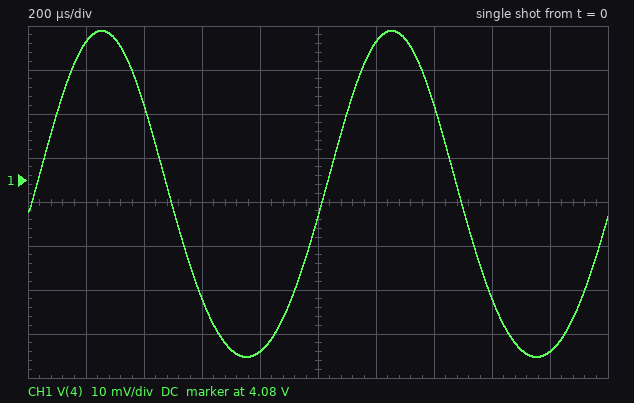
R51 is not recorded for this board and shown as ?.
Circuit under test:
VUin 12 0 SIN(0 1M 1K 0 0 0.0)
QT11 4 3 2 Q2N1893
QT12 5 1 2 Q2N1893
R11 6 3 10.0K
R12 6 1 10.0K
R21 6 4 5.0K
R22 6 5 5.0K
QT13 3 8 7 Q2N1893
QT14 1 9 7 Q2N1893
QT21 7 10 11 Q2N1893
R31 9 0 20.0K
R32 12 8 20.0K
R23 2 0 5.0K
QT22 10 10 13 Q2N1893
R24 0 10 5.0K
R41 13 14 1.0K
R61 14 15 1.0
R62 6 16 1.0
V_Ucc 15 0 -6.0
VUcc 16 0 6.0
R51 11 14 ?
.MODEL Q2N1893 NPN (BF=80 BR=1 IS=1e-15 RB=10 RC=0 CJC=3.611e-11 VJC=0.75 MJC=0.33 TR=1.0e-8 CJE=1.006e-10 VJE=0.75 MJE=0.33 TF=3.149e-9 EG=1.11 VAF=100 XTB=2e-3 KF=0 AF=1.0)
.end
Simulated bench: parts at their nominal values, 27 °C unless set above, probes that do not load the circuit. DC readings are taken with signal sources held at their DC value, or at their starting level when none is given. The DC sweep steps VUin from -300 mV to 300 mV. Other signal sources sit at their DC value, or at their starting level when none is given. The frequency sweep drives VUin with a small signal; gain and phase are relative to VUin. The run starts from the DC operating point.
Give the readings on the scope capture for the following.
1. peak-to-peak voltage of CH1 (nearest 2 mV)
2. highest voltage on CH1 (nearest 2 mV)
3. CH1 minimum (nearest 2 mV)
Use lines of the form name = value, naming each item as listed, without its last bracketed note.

peak-to-peak voltage of CH1 = 74 mV
highest voltage on CH1 = 4.114 V
CH1 minimum = 4.040 V
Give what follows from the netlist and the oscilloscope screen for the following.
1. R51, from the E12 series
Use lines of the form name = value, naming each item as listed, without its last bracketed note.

R51, from the E12 series = 3.3 kΩ
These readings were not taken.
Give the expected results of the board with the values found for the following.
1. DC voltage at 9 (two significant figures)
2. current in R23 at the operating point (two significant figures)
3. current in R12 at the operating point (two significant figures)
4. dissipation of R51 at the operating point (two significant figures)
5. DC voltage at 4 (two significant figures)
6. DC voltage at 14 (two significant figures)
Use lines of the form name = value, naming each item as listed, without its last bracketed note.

DC voltage at 9 = -32 mV
current in R23 at the operating point = 780 µA
current in R12 at the operating point = 140 µA
dissipation of R51 at the operating point = 250 µW
DC voltage at 4 = 4.1 V
DC voltage at 14 = -6.0 V
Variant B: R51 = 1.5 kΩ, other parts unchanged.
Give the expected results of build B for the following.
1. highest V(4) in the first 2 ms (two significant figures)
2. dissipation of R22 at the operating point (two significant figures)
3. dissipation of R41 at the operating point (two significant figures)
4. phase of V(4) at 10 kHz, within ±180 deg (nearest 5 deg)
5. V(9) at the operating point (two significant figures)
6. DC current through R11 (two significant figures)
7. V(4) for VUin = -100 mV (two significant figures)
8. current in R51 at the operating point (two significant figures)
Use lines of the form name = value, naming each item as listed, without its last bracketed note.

highest V(4) in the first 2 ms = 5.1 V
dissipation of R22 at the operating point = 280 µW
dissipation of R41 at the operating point = 770 µW
phase of V(4) at 10 kHz, within ±180 deg = -40 deg
V(9) at the operating point = -70 mV
DC current through R11 = 290 µA
V(4) for VUin = -100 mV = 3.2 V
current in R51 at the operating point = 590 µA
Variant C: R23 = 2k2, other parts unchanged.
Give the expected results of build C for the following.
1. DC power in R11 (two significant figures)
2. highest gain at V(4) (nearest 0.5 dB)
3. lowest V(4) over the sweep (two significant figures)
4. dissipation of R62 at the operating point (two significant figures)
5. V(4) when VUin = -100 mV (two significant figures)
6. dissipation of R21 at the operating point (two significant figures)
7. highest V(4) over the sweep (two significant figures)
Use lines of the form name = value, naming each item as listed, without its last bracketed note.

DC power in R11 = 520 µW
highest gain at V(4) = -11.5 dB
lowest V(4) over the sweep = 2.6 V
dissipation of R62 at the operating point = 2.7 µW
V(4) when VUin = -100 mV = 2.9 V
dissipation of R21 at the operating point = 1.7 mW
highest V(4) over the sweep = 4.8 V
